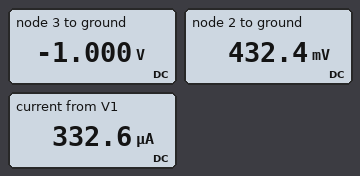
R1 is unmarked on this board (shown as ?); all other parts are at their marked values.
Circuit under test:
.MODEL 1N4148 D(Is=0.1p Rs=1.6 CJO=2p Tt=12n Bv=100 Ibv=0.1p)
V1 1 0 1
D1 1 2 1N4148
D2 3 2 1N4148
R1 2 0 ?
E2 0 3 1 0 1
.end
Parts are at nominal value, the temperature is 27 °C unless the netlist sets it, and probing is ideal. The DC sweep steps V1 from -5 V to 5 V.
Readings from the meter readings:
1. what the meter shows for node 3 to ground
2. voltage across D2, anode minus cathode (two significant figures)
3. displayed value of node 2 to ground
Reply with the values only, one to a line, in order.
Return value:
-1.000 V
-1.4 V
432.4 mV
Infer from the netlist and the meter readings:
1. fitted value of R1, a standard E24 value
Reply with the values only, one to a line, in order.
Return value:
1.3 kΩ
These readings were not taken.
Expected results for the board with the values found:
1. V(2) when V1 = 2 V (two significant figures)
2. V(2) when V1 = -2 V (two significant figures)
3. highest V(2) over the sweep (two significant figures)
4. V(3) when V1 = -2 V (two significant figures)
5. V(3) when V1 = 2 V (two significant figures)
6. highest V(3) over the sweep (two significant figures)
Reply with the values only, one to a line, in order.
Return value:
1.4 V
1.4 V
4.4 V
2.0 V
-2.0 V
5.0 V
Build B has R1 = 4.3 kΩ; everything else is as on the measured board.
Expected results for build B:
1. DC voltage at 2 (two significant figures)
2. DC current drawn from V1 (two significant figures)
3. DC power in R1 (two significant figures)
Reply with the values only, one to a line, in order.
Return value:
460 mV
110 µA
50 µW
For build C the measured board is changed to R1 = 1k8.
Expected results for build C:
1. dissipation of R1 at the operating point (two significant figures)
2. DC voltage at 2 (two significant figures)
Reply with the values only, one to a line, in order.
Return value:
110 µW
440 mV
